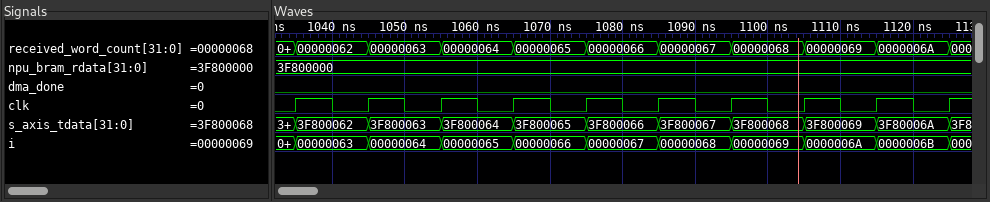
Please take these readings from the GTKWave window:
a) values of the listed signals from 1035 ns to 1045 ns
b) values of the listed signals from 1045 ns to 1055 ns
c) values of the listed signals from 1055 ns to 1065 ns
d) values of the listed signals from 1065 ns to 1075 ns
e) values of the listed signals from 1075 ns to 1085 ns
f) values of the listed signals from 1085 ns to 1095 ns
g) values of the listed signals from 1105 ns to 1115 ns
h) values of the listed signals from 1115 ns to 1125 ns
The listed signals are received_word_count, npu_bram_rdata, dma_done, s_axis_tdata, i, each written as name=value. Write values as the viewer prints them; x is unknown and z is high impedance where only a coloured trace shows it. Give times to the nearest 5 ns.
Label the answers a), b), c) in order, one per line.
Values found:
a) received_word_count=00000062, npu_bram_rdata=3F800000, dma_done=0, s_axis_tdata=3F800062, i=00000063
b) received_word_count=00000063, npu_bram_rdata=3F800000, dma_done=0, s_axis_tdata=3F800063, i=00000064
c) received_word_count=00000064, npu_bram_rdata=3F800000, dma_done=0, s_axis_tdata=3F800064, i=00000065
d) received_word_count=00000065, npu_bram_rdata=3F800000, dma_done=0, s_axis_tdata=3F800065, i=00000066
e) received_word_count=00000066, npu_bram_rdata=3F800000, dma_done=0, s_axis_tdata=3F800066, i=00000067
f) received_word_count=00000067, npu_bram_rdata=3F800000, dma_done=0, s_axis_tdata=3F800067, i=00000068
g) received_word_count=00000069, npu_bram_rdata=3F800000, dma_done=0, s_axis_tdata=3F800069, i=0000006A
h) received_word_count=0000006A, npu_bram_rdata=3F800000, dma_done=0, s_axis_tdata=3F80006A, i=0000006B
